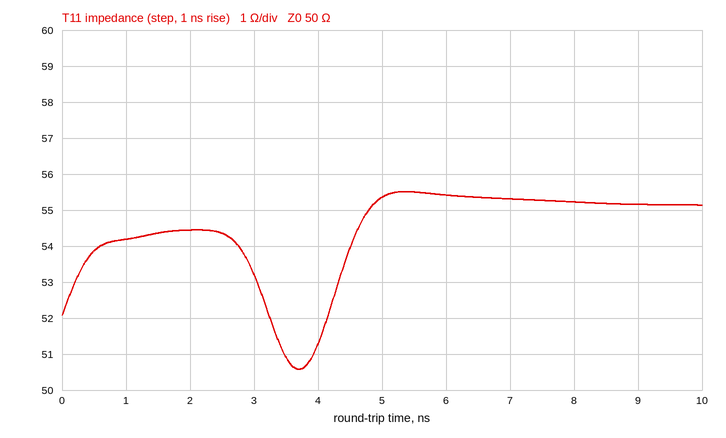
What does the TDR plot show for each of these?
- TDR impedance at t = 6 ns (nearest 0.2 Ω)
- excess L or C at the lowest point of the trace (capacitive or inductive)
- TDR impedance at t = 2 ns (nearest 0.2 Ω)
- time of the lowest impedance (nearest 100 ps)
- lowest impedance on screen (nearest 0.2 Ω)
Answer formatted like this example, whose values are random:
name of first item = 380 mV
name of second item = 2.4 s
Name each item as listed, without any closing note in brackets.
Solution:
TDR impedance at t = 6 ns = 55.4 Ω
excess L or C at the lowest point of the trace = capacitive
TDR impedance at t = 2 ns = 54.4 Ω
time of the lowest impedance = 3.7 ns
lowest impedance on screen = 50.6 Ω
